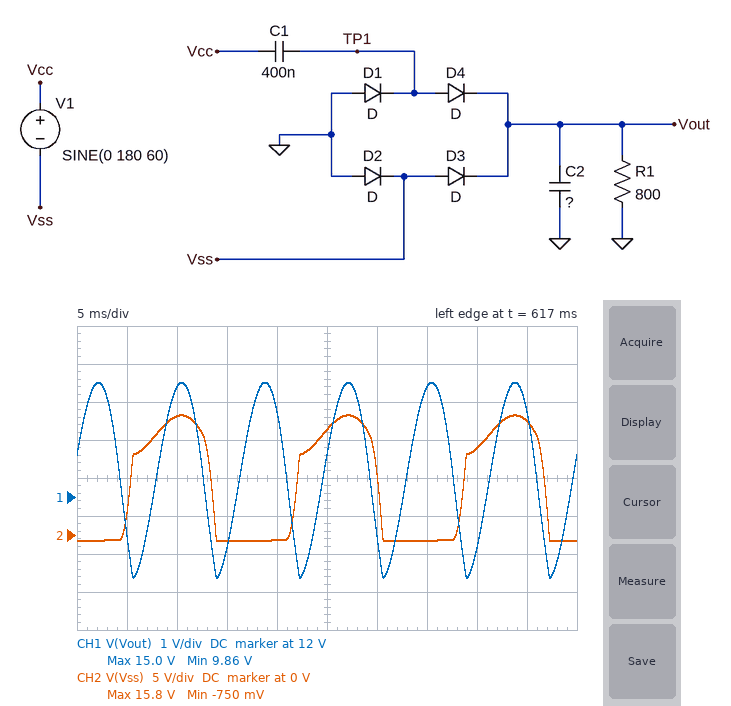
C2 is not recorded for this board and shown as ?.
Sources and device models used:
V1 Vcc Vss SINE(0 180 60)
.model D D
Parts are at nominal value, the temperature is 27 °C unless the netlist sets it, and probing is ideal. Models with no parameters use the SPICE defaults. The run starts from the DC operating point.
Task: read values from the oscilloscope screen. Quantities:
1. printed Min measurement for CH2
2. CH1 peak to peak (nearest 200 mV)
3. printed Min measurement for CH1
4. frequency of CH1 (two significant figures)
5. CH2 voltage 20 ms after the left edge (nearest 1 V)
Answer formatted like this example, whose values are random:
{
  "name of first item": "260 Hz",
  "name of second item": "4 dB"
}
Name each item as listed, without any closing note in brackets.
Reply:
{
  "printed Min measurement for CH2": "-750 mV",
  "CH1 peak to peak": "5.2 V",
  "printed Min measurement for CH1": "9.86 V",
  "frequency of CH1": "120 Hz",
  "CH2 voltage 20 ms after the left edge": "-1 V"
}
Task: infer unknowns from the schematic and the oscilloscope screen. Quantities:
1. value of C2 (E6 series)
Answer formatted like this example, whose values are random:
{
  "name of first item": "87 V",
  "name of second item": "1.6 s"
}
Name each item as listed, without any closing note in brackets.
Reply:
{
  "value of C2": "6.8 µF"
}
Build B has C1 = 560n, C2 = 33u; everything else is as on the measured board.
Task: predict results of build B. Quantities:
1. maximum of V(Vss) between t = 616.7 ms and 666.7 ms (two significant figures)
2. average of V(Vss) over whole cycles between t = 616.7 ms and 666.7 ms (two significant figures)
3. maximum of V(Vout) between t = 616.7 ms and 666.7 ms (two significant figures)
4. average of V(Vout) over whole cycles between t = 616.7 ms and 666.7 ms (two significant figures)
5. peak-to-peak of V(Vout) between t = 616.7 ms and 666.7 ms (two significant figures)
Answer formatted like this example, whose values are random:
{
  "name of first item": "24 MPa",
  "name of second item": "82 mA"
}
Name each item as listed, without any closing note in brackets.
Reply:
{
  "maximum of V(Vss) between t = 616.7 ms and 666.7 ms": "19 V",
  "average of V(Vss) over whole cycles between t = 616.7 ms and 666.7 ms": "8.7 V",
  "maximum of V(Vout) between t = 616.7 ms and 666.7 ms": "18 V",
  "average of V(Vout) over whole cycles between t = 616.7 ms and 666.7 ms": "17 V",
  "peak-to-peak of V(Vout) between t = 616.7 ms and 666.7 ms": "1.6 V"
}
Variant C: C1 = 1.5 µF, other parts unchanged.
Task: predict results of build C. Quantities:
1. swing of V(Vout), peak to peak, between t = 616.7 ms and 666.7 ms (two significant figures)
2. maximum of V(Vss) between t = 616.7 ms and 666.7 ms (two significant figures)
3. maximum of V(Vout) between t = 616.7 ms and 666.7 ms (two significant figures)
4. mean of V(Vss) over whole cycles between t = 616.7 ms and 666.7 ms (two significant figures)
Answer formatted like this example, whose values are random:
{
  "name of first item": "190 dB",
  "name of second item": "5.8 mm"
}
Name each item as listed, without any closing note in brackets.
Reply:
{
  "swing of V(Vout), peak to peak, between t = 616.7 ms and 666.7 ms": "21 V",
  "maximum of V(Vss) between t = 616.7 ms and 666.7 ms": "49 V",
  "maximum of V(Vout) between t = 616.7 ms and 666.7 ms": "48 V",
  "mean of V(Vss) over whole cycles between t = 616.7 ms and 666.7 ms": "20 V"
}
